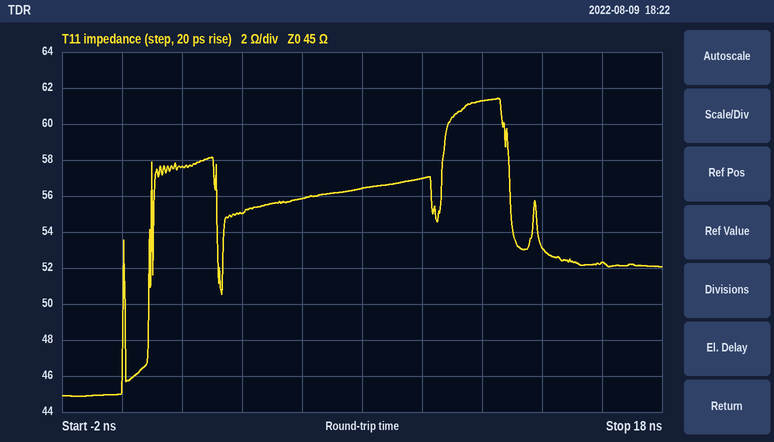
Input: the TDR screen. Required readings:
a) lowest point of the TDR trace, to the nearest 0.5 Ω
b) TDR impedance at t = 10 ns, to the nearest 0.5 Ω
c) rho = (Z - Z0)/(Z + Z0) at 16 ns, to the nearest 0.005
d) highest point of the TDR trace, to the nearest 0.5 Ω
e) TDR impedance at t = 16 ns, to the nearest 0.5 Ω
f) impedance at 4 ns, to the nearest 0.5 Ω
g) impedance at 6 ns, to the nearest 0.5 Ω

45.0 Ω
57.0 Ω
+0.075
61.5 Ω
52.5 Ω
55.0 Ω
56.0 Ω
